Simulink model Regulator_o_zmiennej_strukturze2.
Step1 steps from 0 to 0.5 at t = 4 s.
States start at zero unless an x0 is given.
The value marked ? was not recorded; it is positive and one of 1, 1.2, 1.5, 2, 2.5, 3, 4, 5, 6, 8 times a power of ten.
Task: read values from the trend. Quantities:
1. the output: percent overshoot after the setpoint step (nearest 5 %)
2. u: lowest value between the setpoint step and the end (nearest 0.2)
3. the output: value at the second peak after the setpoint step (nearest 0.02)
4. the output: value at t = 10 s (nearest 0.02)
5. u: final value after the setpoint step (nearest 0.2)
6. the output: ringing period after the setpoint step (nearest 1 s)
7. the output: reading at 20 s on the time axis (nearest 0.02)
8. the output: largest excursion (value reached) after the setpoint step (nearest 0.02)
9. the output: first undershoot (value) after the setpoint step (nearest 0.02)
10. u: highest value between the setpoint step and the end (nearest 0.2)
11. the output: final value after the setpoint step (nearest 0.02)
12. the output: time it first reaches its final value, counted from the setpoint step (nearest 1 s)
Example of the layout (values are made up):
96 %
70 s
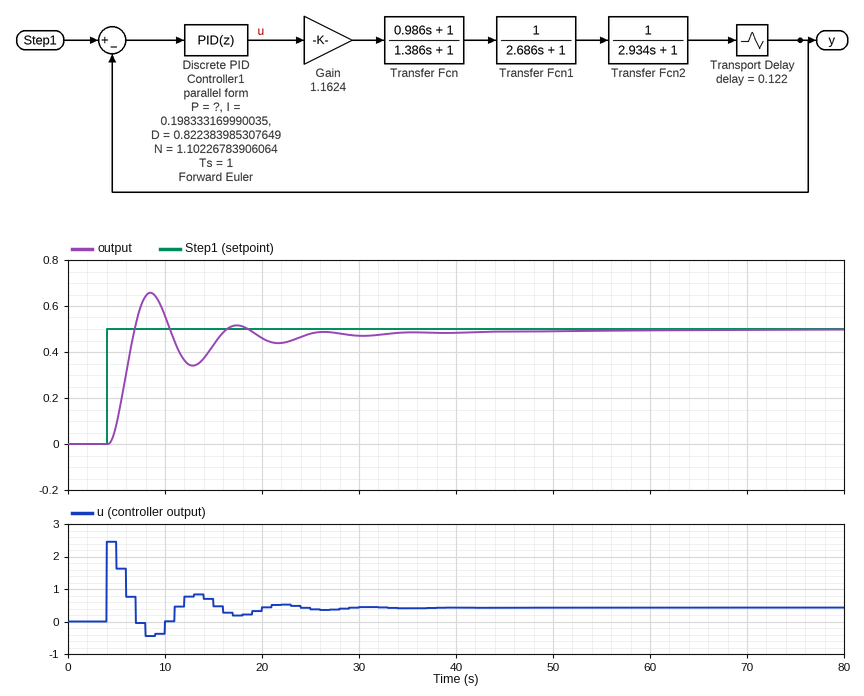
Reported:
30 %
-0.4
0.52
0.56
0.4
9 s
0.46
0.66
0.34
2.4
0.50
3 s
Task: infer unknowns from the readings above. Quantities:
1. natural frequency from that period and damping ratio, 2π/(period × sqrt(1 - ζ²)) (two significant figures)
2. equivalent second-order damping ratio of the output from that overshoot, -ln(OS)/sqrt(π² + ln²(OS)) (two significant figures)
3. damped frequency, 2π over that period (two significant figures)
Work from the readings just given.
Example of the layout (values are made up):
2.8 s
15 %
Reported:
0.75 rad/s
0.36
0.70 rad/s
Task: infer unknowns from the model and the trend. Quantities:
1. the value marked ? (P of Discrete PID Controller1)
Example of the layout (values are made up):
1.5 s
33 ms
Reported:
4
